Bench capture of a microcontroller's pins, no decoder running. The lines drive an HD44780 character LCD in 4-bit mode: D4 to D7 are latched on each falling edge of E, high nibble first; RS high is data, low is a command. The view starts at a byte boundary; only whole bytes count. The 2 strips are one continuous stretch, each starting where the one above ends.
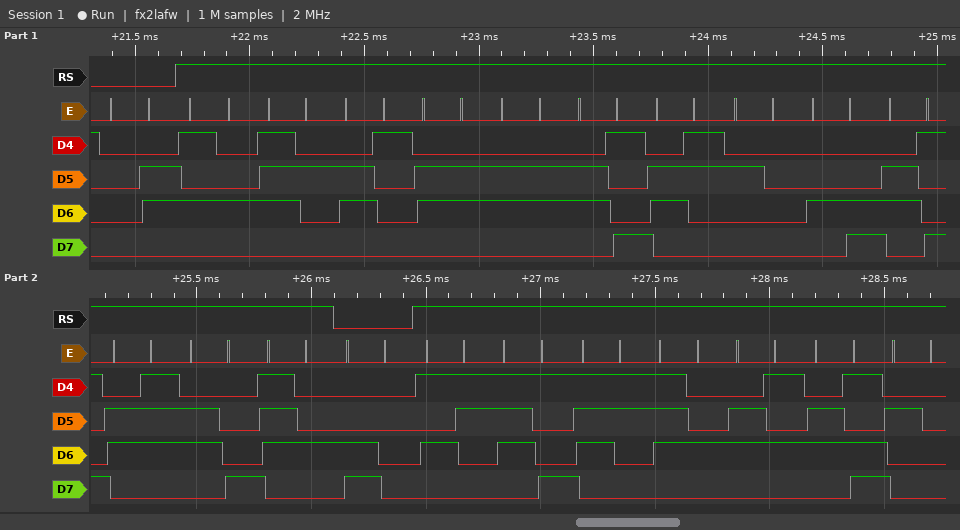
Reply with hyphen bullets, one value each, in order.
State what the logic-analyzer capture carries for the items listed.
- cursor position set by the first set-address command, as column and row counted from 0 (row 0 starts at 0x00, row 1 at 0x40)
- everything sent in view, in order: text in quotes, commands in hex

- column 0, row 1
- 0x06 "Traffic Light" 0xC0 "System "
